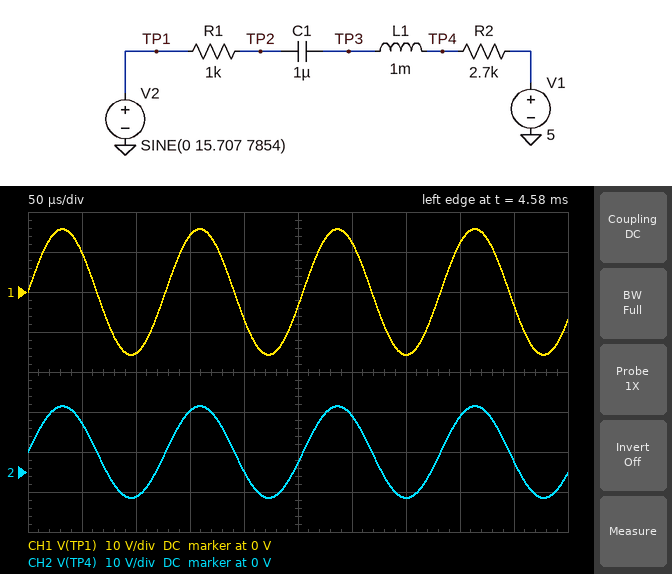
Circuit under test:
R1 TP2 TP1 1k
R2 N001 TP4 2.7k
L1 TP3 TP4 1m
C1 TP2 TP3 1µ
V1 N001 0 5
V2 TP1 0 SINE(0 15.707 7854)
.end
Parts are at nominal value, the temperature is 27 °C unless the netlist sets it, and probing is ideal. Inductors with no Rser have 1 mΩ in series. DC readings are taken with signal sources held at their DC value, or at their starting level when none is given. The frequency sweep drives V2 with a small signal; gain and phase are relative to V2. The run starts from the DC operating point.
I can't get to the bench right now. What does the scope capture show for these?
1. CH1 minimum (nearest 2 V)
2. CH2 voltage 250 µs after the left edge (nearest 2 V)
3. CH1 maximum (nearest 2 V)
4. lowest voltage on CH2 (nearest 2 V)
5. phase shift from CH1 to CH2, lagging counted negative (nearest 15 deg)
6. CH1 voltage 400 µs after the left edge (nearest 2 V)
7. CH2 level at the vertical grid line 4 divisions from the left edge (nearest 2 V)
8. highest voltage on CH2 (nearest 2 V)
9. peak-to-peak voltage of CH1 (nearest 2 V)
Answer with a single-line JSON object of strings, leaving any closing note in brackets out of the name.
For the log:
{"CH1 minimum": "-16 V", "CH2 voltage 250 µs after the left edge": "2 V", "CH1 maximum": "16 V", "lowest voltage on CH2": "-6 V", "phase shift from CH1 to CH2, lagging counted negative": "0 deg", "CH1 voltage 400 µs after the left edge": "12 V", "CH2 level at the vertical grid line 4 divisions from the left edge": "0 V", "highest voltage on CH2": "16 V", "peak-to-peak voltage of CH1": "32 V"}
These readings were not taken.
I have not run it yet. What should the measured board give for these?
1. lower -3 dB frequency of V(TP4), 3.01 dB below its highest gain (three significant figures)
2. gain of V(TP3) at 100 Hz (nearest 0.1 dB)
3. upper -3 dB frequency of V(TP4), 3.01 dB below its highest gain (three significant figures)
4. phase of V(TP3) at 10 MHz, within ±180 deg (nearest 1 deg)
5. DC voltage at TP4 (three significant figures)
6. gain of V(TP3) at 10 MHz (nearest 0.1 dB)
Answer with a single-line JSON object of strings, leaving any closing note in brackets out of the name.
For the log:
{"lower -3 dB frequency of V(TP4), 3.01 dB below its highest gain": "43.0 Hz", "gain of V(TP3) at 100 Hz": "-3.5 dB", "upper -3 dB frequency of V(TP4), 3.01 dB below its highest gain": "589 kHz", "phase of V(TP3) at 10 MHz, within ±180 deg": "1 deg", "DC voltage at TP4": "5.00 V", "gain of V(TP3) at 10 MHz": "0 dB"}
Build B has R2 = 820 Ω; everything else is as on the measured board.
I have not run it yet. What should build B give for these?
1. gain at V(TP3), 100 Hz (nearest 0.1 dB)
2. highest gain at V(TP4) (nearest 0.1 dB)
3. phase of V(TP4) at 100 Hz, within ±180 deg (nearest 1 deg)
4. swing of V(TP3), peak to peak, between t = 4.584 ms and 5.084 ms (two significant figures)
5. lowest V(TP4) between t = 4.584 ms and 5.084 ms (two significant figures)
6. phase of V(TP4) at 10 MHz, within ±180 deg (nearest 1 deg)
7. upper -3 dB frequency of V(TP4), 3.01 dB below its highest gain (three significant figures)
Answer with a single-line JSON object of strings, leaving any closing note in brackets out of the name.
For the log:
{"gain at V(TP3), 100 Hz": "-9.4 dB", "highest gain at V(TP4)": "-6.9 dB", "phase of V(TP4) at 100 Hz, within ±180 deg": "41 deg", "swing of V(TP3), peak to peak, between t = 4.584 ms and 5.084 ms": "14 V", "lowest V(TP4) between t = 4.584 ms and 5.084 ms": "-2.1 V", "phase of V(TP4) at 10 MHz, within ±180 deg": "-88 deg", "upper -3 dB frequency of V(TP4), 3.01 dB below its highest gain": "290 kHz"}
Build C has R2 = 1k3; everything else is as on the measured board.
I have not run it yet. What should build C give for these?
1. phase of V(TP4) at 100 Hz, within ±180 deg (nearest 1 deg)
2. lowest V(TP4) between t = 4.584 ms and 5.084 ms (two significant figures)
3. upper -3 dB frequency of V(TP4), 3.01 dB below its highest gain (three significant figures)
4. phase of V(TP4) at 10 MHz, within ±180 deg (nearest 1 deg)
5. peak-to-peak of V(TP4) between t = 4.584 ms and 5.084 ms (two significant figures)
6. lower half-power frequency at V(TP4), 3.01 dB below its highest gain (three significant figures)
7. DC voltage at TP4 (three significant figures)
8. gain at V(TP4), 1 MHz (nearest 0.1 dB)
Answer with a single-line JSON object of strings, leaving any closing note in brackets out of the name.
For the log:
{"phase of V(TP4) at 100 Hz, within ±180 deg": "35 deg", "lowest V(TP4) between t = 4.584 ms and 5.084 ms": "-3.9 V", "upper -3 dB frequency of V(TP4), 3.01 dB below its highest gain": "366 kHz", "phase of V(TP4) at 10 MHz, within ±180 deg": "-88 deg", "peak-to-peak of V(TP4) between t = 4.584 ms and 5.084 ms": "18 V", "lower half-power frequency at V(TP4), 3.01 dB below its highest gain": "69.2 Hz", "DC voltage at TP4": "5.00 V", "gain at V(TP4), 1 MHz": "-14.2 dB"}
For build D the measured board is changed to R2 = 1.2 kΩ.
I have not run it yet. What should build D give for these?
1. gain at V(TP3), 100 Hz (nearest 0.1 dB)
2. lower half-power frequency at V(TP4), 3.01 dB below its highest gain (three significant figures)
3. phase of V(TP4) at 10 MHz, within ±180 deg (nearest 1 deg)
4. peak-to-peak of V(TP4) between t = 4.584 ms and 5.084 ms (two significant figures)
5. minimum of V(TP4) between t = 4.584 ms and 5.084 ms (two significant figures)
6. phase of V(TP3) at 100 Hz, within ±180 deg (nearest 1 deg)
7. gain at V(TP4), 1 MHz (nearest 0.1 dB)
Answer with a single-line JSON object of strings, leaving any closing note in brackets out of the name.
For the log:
{"gain at V(TP3), 100 Hz": "-7.1 dB", "lower half-power frequency at V(TP4), 3.01 dB below its highest gain": "72.3 Hz", "phase of V(TP4) at 10 MHz, within ±180 deg": "-88 deg", "peak-to-peak of V(TP4) between t = 4.584 ms and 5.084 ms": "17 V", "minimum of V(TP4) between t = 4.584 ms and 5.084 ms": "-3.6 V", "phase of V(TP3) at 100 Hz, within ±180 deg": "36 deg", "gain at V(TP4), 1 MHz": "-14.9 dB"}
